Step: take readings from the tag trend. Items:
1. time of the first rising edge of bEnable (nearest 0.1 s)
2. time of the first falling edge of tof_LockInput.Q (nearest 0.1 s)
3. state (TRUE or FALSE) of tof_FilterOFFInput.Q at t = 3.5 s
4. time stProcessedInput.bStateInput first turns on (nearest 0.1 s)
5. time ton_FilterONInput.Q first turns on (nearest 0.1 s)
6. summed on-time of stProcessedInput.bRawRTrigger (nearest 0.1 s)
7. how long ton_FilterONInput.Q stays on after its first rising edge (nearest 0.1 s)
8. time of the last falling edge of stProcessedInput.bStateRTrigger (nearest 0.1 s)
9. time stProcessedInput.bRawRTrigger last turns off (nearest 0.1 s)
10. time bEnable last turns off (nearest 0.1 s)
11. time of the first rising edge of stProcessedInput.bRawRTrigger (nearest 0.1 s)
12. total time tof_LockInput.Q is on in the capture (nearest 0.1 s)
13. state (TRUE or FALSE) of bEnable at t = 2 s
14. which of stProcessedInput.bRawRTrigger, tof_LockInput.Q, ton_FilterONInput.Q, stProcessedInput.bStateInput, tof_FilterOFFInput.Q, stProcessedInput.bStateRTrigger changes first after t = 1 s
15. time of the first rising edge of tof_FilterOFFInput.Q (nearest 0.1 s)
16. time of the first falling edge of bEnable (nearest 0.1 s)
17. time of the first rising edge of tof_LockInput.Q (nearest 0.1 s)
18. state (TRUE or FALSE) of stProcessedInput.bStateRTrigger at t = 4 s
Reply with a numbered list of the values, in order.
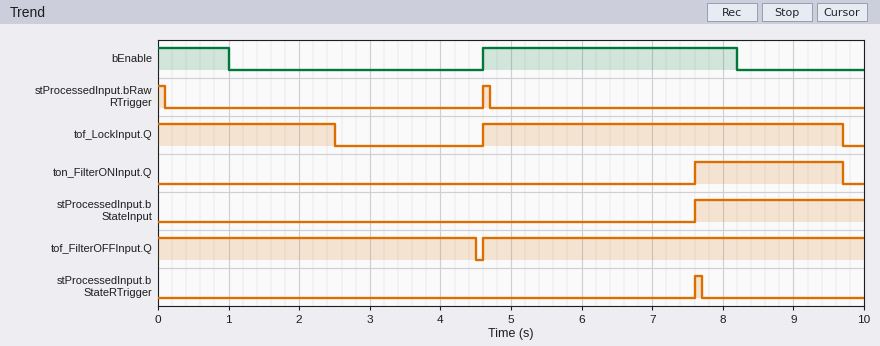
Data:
1. 4.6 s
2. 2.5 s
3. TRUE
4. 7.6 s
5. 7.6 s
6. 0.2 s
7. 2.1 s
8. 7.7 s
9. 4.7 s
10. 8.2 s
11. 4.6 s
12. 7.6 s
13. FALSE
14. tof_LockInput.Q
15. 4.6 s
16. 1.0 s
17. 4.6 s
18. FALSE
